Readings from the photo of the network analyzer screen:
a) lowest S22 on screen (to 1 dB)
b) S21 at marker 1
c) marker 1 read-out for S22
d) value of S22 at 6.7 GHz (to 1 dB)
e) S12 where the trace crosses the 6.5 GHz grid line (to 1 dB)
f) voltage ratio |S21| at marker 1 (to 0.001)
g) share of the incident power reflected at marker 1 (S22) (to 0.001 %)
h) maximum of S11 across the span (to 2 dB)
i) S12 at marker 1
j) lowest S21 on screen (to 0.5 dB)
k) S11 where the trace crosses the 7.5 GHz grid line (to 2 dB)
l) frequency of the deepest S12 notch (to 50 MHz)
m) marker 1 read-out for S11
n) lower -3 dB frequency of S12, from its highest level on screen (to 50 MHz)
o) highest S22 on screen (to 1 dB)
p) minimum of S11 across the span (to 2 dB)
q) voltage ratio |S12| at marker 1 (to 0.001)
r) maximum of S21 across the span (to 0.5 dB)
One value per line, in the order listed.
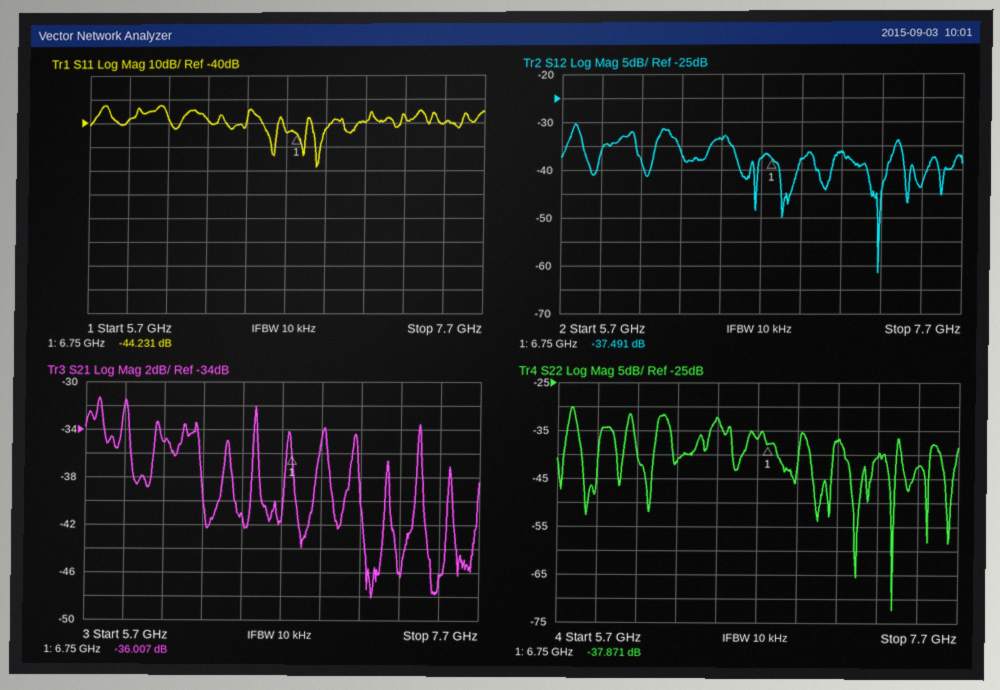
-72 dB
-36.007 dB
-37.871 dB
-37 dB
-34 dB
0.016
0.016 %
-32 dB
-37.491 dB
-48.0 dB
-40 dB
7.30 GHz
-44.231 dB
5.75 GHz
-30 dB
-58 dB
0.013
-31.5 dB
